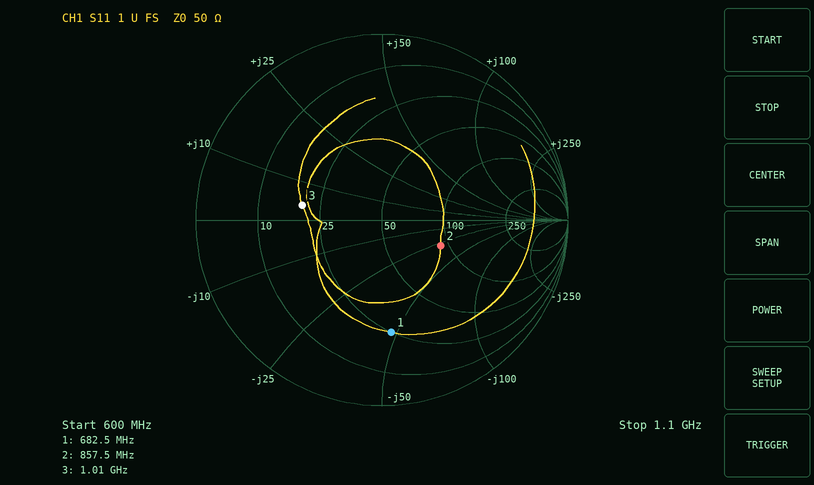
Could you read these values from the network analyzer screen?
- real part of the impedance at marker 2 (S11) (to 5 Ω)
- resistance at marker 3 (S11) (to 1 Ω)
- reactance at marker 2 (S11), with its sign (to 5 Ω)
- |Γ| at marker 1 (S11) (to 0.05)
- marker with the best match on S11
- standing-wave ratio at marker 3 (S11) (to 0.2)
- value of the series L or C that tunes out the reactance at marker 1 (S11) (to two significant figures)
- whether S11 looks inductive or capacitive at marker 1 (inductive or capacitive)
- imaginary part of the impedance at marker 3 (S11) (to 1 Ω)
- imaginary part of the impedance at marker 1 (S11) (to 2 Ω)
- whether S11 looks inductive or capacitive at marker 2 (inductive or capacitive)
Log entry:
90 Ω
20 Ω
-30 Ω
0.60
marker 2
2.6
11 nH
capacitive
+4 Ω
-48 Ω
capacitive
